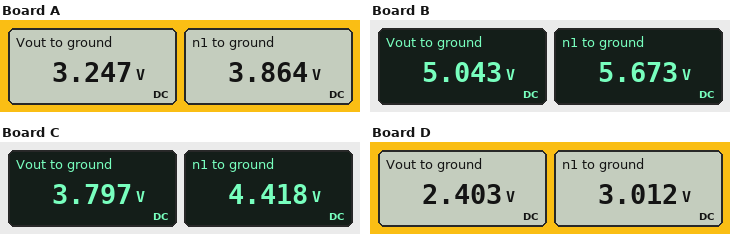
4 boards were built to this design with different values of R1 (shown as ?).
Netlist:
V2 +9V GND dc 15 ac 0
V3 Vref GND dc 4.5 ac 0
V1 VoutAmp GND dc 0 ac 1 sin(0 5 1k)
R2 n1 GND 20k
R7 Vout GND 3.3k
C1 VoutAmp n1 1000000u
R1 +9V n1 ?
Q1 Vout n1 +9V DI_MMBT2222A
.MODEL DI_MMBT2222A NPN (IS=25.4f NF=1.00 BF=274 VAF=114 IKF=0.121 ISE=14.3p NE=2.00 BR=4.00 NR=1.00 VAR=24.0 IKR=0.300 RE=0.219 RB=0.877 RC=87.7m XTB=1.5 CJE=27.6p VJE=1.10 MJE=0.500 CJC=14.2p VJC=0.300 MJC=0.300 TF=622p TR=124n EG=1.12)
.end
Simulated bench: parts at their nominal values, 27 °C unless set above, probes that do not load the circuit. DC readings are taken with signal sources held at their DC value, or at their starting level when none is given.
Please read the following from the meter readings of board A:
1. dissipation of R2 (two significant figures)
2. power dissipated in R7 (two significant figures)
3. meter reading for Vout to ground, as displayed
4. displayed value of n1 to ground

750 µW
3.2 mW
3.247 V
3.864 V
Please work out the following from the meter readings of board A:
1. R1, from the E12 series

33 kΩ
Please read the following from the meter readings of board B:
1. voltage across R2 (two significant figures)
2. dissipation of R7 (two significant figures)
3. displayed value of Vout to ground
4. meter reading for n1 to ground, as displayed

5.7 V
7.7 mW
5.043 V
5.673 V
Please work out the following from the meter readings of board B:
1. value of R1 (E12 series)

18 kΩ
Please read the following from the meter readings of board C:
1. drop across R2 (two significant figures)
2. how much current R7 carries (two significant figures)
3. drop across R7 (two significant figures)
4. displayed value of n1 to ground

4.4 V
1.2 mA
3.8 V
4.418 V
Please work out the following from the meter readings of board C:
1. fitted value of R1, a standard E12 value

27 kΩ
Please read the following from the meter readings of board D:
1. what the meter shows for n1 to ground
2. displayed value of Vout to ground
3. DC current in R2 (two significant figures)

3.012 V
2.403 V
150 µA
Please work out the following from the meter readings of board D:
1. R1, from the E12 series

47 kΩ
